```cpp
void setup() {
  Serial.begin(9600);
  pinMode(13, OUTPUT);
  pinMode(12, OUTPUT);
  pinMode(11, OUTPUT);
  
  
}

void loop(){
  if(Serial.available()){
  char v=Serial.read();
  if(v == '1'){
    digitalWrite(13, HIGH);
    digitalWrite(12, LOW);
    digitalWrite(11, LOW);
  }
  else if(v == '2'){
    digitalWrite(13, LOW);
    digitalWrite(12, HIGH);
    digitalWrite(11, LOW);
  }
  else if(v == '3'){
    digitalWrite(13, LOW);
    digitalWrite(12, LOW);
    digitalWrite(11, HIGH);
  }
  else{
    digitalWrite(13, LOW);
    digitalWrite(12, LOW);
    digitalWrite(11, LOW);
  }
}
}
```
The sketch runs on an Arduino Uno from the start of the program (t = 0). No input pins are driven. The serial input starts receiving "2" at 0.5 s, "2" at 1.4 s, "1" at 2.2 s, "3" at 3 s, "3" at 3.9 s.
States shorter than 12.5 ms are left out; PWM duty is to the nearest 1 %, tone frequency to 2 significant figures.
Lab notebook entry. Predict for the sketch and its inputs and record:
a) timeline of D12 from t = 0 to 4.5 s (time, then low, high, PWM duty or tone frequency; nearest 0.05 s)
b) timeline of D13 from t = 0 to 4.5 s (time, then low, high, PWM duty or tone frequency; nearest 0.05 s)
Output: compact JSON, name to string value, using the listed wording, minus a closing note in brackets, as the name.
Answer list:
{"timeline of D12 from t = 0 to 4.5 s": "0 s low; 0.5 s high; 2.2 s low", "timeline of D13 from t = 0 to 4.5 s": "0 s low; 2.2 s high; 3 s low"}
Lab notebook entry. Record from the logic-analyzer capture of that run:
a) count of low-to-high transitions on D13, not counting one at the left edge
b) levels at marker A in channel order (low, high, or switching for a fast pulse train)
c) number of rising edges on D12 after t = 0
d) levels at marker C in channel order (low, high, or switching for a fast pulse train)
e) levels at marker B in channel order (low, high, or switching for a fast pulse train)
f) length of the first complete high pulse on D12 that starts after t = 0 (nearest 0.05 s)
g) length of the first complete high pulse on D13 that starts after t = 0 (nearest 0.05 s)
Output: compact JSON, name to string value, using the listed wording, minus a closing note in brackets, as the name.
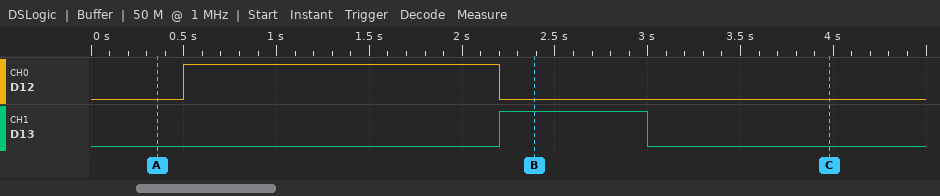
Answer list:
{"count of low-to-high transitions on D13, not counting one at the left edge": "1", "levels at marker A in channel order": "D12 low, D13 low", "number of rising edges on D12 after t = 0": "1", "levels at marker C in channel order": "D12 low, D13 low", "levels at marker B in channel order": "D12 low, D13 high", "length of the first complete high pulse on D12 that starts after t = 0": "1.70 s", "length of the first complete high pulse on D13 that starts after t = 0": "0.80 s"}
